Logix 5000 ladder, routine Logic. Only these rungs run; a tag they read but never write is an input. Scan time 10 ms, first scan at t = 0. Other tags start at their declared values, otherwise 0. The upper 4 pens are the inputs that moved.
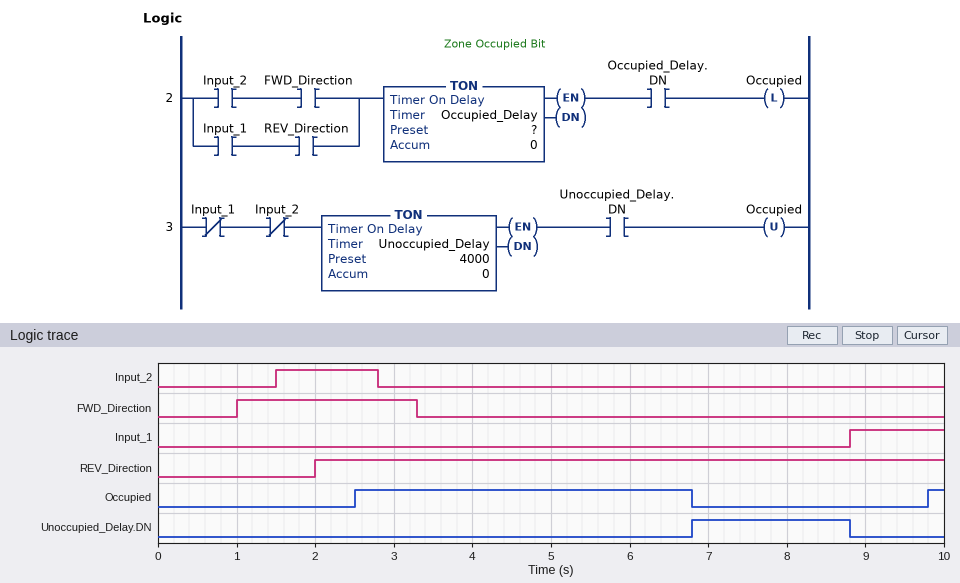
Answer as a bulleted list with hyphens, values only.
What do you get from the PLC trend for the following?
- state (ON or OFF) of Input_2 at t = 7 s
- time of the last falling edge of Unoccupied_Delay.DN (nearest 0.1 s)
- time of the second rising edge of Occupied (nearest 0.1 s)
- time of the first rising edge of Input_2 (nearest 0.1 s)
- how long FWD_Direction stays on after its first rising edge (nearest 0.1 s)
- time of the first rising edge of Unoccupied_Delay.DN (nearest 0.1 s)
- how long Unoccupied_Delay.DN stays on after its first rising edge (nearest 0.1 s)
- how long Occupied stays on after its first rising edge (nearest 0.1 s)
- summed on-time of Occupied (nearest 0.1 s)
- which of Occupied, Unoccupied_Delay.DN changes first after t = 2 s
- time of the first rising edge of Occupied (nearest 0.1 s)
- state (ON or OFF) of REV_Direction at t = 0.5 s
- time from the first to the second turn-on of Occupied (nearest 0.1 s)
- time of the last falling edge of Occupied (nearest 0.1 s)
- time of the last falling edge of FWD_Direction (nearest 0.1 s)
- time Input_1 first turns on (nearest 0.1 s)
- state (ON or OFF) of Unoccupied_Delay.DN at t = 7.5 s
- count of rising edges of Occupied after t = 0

- OFF
- 8.8 s
- 9.8 s
- 1.5 s
- 2.3 s
- 6.8 s
- 2.0 s
- 4.3 s
- 4.5 s
- Occupied
- 2.5 s
- OFF
- 7.3 s
- 6.8 s
- 3.3 s
- 8.8 s
- ON
- 2
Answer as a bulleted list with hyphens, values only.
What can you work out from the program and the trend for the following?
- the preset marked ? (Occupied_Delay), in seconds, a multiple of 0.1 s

- 1.0 s
